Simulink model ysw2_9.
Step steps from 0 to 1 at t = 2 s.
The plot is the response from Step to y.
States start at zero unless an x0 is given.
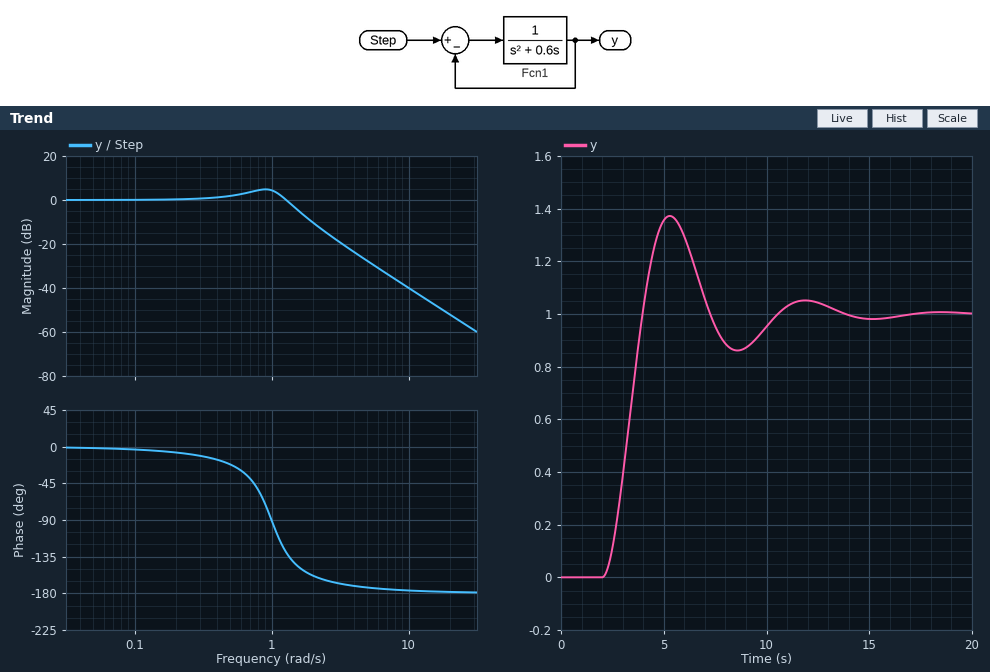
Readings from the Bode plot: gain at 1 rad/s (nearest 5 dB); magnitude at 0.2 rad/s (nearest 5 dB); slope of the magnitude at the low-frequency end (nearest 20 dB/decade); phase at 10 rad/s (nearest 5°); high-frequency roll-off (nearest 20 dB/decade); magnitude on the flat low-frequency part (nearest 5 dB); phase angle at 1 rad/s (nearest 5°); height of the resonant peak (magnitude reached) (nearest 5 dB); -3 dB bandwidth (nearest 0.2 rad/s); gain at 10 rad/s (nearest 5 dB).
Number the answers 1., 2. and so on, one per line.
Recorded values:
1. 5 dB
2. 0 dB
3. 0 dB/decade
4. -175°
5. -40 dB/decade
6. 0 dB
7. -90°
8. 5 dB
9. 1.4 rad/s
10. -40 dB
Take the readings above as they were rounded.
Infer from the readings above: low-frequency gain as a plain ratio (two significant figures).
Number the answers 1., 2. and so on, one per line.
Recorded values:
1. 1.0
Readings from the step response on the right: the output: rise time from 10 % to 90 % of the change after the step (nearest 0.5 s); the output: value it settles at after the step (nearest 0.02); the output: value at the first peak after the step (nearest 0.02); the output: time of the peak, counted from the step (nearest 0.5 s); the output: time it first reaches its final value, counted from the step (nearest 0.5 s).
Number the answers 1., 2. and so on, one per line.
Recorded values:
1. 1.5 s
2. 1.00
3. 1.38
4. 3.5 s
5. 2.0 s
